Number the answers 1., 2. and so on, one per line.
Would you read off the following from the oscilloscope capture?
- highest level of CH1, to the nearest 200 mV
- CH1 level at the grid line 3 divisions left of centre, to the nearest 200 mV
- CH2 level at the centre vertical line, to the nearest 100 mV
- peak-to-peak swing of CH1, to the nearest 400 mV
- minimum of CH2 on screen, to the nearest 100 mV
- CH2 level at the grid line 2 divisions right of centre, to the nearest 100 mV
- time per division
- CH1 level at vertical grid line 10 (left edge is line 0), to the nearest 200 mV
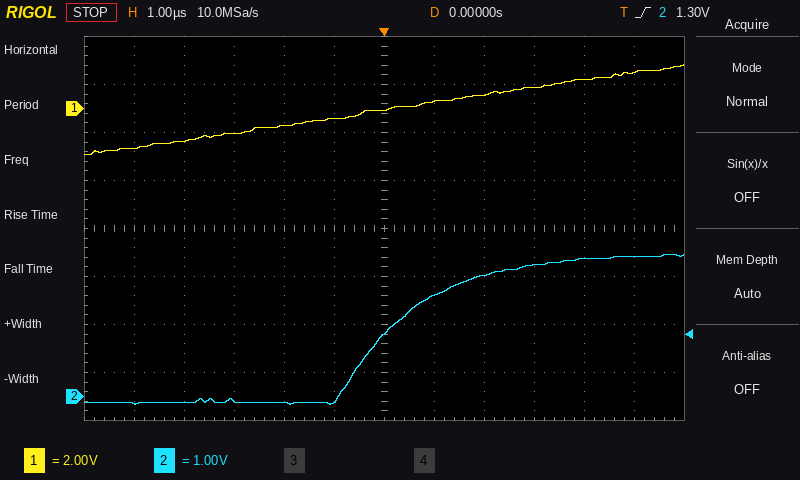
1. 1.8 V
2. -1.0 V
3. 1.3 V
4. 3.6 V
5. -200 mV
6. 2.5 V
7. 1 µs
8. 1.2 V
